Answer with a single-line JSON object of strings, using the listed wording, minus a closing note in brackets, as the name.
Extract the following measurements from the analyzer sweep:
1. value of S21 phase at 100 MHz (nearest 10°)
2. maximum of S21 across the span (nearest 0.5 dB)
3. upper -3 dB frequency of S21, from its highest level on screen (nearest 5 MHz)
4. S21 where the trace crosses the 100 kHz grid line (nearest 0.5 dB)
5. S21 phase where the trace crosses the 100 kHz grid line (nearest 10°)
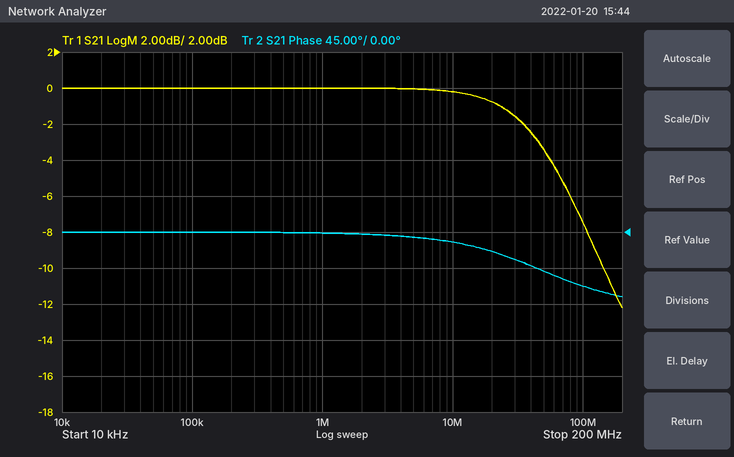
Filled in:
{"value of S21 phase at 100 MHz": "-70°", "maximum of S21 across the span": "0.0 dB", "upper -3 dB frequency of S21, from its highest level on screen": "45 MHz", "S21 where the trace crosses the 100 kHz grid line": "0.0 dB", "S21 phase where the trace crosses the 100 kHz grid line": "0°"}
